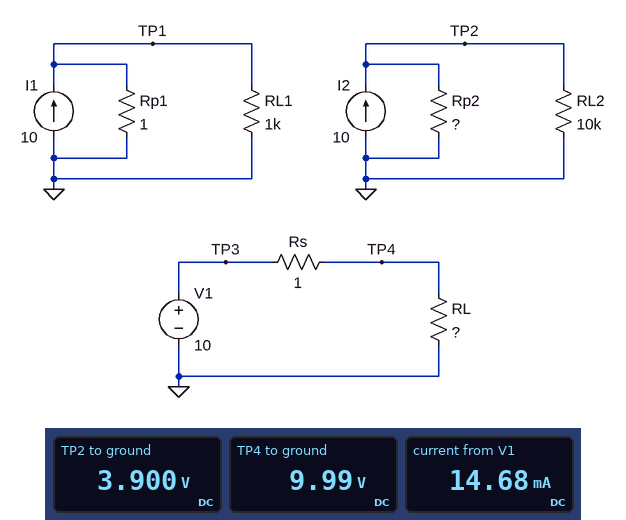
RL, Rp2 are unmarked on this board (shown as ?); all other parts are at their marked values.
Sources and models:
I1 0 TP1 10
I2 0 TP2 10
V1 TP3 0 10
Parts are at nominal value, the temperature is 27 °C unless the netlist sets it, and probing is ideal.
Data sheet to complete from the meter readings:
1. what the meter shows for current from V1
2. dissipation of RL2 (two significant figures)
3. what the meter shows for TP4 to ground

14.68 mA
1.5 mW
9.99 V
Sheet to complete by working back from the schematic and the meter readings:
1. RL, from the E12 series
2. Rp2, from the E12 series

680 Ω
0.39 Ω
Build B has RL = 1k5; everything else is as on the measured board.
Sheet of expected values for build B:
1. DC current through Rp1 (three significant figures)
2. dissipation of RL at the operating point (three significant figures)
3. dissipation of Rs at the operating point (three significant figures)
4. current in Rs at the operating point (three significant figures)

9.99 A
66.6 mW
44.4 µW
6.66 mA
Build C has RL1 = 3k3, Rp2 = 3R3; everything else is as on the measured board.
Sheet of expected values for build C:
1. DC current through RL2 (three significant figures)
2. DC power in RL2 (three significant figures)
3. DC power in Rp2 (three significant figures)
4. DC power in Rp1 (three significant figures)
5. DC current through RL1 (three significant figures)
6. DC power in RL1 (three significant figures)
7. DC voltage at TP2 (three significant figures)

3.30 mA
109 mW
330 W
99.9 W
3.03 mA
30.3 mW
33.0 V
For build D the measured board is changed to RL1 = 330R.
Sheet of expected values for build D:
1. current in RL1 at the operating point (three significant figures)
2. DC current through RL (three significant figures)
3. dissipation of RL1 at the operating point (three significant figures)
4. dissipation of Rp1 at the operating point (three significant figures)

30.2 mA
14.7 mA
301 mW
99.4 W
